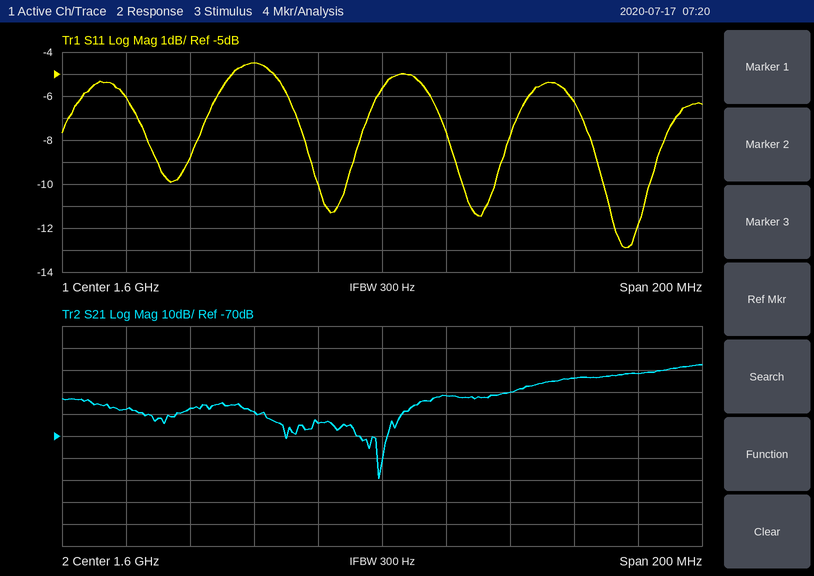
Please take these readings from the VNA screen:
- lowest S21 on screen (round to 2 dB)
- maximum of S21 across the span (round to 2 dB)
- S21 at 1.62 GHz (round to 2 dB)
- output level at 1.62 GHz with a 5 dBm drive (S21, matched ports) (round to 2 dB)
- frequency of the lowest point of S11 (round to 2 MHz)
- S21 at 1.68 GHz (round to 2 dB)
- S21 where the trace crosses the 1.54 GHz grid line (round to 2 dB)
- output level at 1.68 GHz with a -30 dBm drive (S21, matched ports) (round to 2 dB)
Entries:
-90 dB
-38 dB
-52 dB
-46 dBm
1.676 GHz
-42 dB
-58 dB
-72 dBm
